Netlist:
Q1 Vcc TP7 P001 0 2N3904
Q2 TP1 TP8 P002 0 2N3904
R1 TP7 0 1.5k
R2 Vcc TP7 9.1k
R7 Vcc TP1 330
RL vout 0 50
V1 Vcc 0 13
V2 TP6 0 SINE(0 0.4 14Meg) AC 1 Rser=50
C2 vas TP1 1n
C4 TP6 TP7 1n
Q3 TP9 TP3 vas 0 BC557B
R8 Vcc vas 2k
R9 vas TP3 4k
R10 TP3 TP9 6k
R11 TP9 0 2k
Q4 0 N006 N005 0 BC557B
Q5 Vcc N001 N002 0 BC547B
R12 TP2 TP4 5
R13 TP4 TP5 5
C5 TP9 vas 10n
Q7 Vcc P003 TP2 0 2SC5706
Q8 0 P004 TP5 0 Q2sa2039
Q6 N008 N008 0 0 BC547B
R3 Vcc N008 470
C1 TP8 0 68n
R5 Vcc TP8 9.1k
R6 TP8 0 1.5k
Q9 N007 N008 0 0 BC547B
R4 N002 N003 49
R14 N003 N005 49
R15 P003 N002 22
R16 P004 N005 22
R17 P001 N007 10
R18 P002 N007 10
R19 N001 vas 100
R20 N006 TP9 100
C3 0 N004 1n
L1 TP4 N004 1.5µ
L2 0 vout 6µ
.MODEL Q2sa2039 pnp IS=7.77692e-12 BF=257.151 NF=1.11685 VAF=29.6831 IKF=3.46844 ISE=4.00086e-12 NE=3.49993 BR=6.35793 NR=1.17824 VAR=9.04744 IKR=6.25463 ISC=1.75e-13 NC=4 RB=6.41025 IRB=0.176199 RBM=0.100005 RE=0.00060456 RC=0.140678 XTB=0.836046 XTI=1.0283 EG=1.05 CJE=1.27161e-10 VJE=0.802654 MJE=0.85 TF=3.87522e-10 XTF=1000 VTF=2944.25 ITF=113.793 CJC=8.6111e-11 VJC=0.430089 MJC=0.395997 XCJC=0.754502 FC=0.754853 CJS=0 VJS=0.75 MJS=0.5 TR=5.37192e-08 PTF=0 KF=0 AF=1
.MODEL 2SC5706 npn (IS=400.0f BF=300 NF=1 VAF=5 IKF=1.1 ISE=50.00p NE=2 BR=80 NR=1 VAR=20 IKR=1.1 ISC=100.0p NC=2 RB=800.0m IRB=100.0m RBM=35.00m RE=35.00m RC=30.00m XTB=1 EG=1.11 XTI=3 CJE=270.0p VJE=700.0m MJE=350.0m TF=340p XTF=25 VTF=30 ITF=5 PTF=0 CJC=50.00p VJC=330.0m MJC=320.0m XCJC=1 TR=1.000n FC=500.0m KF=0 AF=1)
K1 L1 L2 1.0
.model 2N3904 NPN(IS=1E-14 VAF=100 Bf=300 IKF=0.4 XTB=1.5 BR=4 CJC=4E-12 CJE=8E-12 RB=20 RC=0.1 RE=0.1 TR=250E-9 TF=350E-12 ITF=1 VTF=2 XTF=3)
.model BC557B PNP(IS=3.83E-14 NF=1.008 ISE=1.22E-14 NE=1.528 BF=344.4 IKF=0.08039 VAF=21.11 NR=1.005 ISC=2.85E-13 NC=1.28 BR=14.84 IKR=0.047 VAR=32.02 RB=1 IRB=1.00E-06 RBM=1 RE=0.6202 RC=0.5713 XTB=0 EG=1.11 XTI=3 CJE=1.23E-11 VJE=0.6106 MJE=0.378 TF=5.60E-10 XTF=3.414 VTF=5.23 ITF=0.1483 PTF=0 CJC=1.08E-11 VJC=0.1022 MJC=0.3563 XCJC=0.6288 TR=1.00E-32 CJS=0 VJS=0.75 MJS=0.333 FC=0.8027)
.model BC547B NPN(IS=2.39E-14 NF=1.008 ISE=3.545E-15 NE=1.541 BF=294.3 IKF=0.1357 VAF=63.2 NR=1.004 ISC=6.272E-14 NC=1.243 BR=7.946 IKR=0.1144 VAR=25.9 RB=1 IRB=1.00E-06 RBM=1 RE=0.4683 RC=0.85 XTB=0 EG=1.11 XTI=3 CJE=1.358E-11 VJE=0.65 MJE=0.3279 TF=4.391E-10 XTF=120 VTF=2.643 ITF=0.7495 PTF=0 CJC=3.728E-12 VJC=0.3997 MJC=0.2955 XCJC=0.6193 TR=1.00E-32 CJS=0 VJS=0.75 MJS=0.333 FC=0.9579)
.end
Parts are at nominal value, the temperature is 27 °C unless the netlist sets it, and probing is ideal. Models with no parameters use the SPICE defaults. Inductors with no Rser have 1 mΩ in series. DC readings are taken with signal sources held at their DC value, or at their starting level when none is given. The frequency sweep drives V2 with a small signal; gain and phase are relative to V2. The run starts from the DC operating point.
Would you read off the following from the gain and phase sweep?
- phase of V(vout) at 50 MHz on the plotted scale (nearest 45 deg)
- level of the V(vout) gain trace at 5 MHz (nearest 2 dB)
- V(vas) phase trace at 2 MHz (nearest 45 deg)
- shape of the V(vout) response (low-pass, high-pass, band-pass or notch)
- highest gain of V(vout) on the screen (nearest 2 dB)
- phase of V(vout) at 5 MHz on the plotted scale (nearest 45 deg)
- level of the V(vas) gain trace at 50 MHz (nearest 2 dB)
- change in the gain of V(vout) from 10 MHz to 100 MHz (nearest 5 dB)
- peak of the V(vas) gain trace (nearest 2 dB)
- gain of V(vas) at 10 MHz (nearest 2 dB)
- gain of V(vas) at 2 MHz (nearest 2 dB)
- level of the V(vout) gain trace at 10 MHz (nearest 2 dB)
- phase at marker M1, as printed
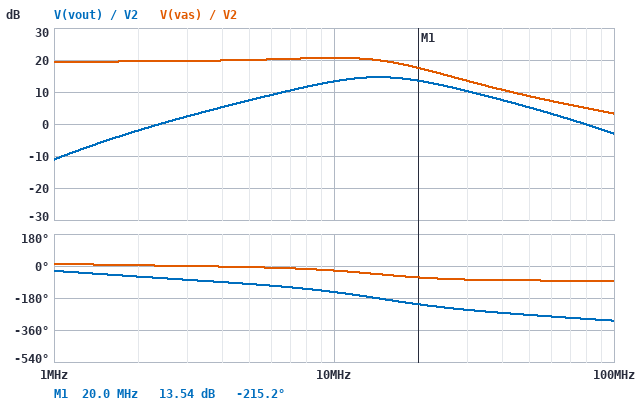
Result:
-270 deg
8 dB
0 deg
band-pass
14 dB
-90 deg
8 dB
-15 dB
20 dB
20 dB
20 dB
14 dB
-215.2 deg
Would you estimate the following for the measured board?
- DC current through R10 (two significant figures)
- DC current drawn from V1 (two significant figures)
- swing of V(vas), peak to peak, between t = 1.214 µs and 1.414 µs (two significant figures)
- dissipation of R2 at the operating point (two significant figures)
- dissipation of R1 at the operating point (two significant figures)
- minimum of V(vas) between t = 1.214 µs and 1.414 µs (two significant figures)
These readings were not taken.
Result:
170 µA
61 mA
8.3 V
14 mW
2.1 mW
3.3 V
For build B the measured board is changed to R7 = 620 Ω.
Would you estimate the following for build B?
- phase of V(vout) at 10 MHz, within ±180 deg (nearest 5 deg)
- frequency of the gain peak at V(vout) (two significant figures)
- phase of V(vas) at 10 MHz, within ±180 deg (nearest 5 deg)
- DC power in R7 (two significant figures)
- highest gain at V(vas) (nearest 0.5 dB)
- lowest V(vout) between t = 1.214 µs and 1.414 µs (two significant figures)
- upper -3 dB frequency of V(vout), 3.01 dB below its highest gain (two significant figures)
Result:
-160 deg
12 MHz
-40 deg
100 mW
24.5 dB
-7.8 V
20 MHz
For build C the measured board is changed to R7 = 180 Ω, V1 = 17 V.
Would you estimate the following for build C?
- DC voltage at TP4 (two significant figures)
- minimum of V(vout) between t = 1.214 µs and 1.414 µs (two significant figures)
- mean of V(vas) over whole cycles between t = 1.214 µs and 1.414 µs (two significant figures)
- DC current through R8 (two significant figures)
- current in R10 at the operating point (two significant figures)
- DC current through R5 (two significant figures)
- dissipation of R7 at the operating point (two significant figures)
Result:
8.5 V
-4.0 V
9.3 V
3.8 mA
180 µA
1.6 mA
53 mW
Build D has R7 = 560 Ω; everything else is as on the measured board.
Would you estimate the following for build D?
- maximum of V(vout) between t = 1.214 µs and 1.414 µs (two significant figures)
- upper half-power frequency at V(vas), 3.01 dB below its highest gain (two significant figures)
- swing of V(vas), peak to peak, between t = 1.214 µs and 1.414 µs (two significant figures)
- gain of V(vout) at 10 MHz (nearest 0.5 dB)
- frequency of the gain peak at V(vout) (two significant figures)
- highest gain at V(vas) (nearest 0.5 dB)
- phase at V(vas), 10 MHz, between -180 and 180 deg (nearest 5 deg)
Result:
7.5 V
16 MHz
11 V
16.5 dB
12 MHz
24.0 dB
-35 deg
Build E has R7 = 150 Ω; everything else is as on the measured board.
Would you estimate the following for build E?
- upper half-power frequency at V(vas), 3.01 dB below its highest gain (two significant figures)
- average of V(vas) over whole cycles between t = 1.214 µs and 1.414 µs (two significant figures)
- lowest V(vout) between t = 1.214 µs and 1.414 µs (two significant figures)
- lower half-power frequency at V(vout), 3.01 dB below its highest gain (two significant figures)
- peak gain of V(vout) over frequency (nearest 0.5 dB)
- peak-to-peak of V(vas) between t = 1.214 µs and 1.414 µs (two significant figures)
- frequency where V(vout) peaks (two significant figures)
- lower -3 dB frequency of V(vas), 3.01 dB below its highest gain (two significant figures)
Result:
28 MHz
7.3 V
-2.8 V
9.2 MHz
9.5 dB
4.2 V
18 MHz
250 kHz
